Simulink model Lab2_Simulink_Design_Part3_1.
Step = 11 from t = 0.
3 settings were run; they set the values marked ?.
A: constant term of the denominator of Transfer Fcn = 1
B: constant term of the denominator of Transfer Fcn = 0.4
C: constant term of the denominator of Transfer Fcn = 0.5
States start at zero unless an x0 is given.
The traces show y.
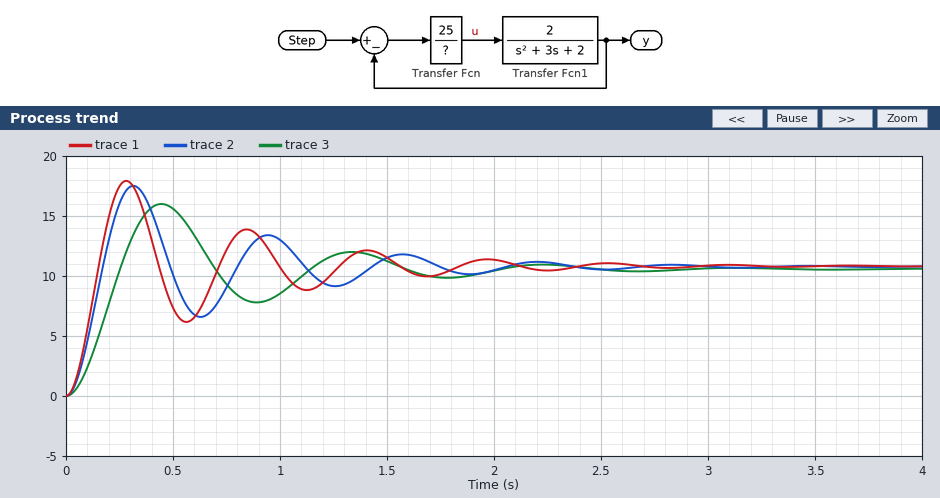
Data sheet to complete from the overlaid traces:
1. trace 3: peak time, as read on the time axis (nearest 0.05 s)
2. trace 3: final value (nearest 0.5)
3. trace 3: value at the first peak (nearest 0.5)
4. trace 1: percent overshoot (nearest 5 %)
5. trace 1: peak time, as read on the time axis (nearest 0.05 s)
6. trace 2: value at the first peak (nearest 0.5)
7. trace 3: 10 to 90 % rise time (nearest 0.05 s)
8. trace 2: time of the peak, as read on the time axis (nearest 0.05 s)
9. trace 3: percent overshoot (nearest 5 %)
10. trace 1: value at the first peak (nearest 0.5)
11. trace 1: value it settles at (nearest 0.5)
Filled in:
0.45 s
10.5
16.0
65 %
0.30 s
17.5
0.15 s
0.30 s
50 %
18.0
11.0
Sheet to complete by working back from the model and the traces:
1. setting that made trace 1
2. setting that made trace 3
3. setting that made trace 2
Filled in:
B
A
C
